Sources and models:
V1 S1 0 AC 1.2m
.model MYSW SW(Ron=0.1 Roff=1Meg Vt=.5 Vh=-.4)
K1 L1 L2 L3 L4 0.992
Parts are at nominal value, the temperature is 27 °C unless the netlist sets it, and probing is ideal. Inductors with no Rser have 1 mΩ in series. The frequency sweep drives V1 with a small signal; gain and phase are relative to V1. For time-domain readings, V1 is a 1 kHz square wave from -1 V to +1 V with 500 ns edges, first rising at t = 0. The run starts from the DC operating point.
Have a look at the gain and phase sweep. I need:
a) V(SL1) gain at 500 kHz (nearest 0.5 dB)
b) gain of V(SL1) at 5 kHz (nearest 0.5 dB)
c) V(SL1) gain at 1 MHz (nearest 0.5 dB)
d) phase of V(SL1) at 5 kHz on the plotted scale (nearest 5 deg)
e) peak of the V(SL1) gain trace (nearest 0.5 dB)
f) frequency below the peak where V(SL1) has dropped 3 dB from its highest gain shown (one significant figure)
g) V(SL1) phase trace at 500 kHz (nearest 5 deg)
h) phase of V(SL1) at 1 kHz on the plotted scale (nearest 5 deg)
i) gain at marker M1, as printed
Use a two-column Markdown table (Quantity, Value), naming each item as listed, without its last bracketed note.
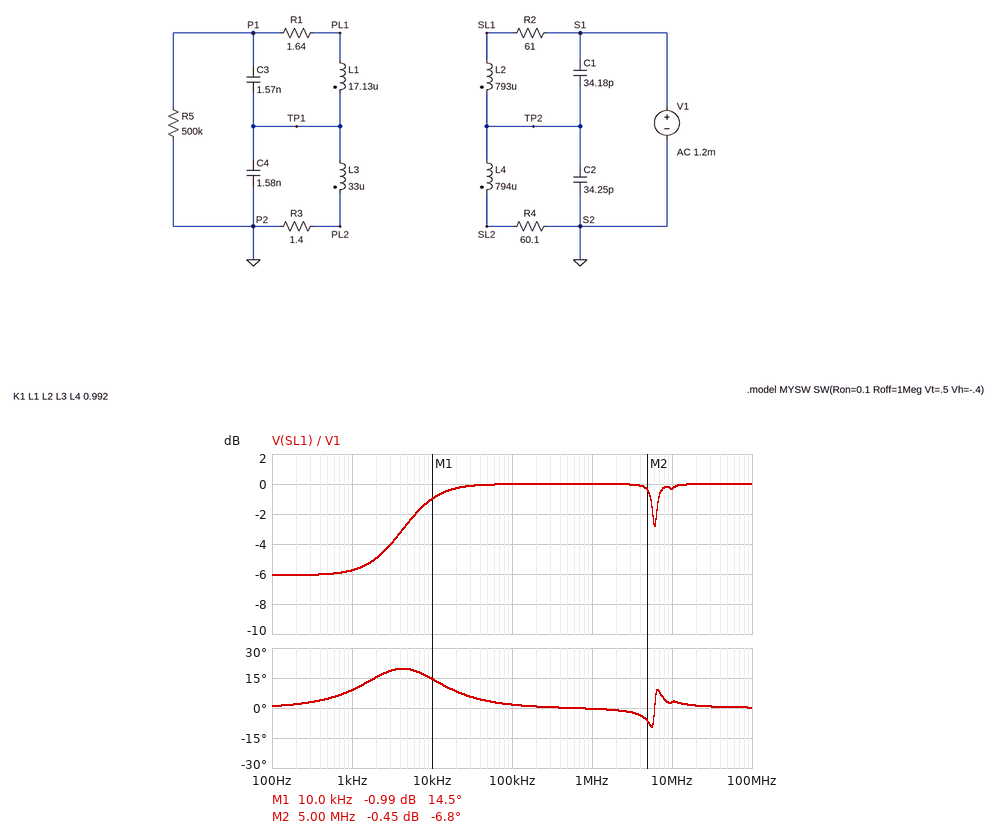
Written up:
| Quantity | Value |
|---|---|
| V(SL1) gain at 500 kHz | 0 dB |
| gain of V(SL1) at 5 kHz | -2.5 dB |
| V(SL1) gain at 1 MHz | 0 dB |
| phase of V(SL1) at 5 kHz on the plotted scale | 20 deg |
| peak of the V(SL1) gain trace | 0 dB |
| frequency below the peak where V(SL1) has dropped 3 dB from its highest gain shown | 4 kHz |
| V(SL1) phase trace at 500 kHz | 0 deg |
| phase of V(SL1) at 1 kHz on the plotted scale | 10 deg |
| gain at marker M1, as printed | -0.99 dB |
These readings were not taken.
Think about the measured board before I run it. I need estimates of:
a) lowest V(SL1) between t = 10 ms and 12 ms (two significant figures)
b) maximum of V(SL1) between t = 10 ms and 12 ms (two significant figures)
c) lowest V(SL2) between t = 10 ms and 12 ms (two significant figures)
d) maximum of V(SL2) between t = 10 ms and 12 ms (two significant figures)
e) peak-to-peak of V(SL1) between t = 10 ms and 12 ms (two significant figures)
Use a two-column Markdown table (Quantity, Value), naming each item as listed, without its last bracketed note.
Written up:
| Quantity | Value |
|---|---|
| lowest V(SL1) between t = 10 ms and 12 ms | -1.5 V |
| maximum of V(SL1) between t = 10 ms and 12 ms | 1.5 V |
| lowest V(SL2) between t = 10 ms and 12 ms | -500 mV |
| maximum of V(SL2) between t = 10 ms and 12 ms | 500 mV |
| peak-to-peak of V(SL1) between t = 10 ms and 12 ms | 3.0 V |
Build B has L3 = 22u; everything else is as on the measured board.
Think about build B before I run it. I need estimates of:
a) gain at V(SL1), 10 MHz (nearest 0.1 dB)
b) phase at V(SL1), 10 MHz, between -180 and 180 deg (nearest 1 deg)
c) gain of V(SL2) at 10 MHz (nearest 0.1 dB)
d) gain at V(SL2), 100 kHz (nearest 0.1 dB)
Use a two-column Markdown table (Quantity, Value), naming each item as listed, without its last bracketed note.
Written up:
| Quantity | Value |
|---|---|
| gain at V(SL1), 10 MHz | -0.2 dB |
| phase at V(SL1), 10 MHz, between -180 and 180 deg | 4 deg |
| gain of V(SL2) at 10 MHz | -23.3 dB |
| gain at V(SL2), 100 kHz | -30.6 dB |
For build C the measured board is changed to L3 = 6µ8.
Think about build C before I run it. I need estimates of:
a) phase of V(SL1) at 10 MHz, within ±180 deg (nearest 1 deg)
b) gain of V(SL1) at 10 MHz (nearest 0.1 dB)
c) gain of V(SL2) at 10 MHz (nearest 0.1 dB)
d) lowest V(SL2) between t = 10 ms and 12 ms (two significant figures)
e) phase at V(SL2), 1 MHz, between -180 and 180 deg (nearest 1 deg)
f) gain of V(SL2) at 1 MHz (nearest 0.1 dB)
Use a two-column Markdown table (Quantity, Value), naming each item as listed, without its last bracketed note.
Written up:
| Quantity | Value |
|---|---|
| phase of V(SL1) at 10 MHz, within ±180 deg | 5 deg |
| gain of V(SL1) at 10 MHz | -0.5 dB |
| gain of V(SL2) at 10 MHz | -20.6 dB |
| lowest V(SL2) between t = 10 ms and 12 ms | -500 mV |
| phase at V(SL2), 1 MHz, between -180 and 180 deg | 87 deg |
| gain of V(SL2) at 1 MHz | -56.7 dB |
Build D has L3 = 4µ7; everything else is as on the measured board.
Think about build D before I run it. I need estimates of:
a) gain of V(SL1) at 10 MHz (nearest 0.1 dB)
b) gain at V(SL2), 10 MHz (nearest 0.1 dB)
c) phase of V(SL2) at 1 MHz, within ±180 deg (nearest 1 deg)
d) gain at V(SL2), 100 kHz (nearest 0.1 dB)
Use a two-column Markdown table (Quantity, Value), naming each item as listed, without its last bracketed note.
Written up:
| Quantity | Value |
|---|---|
| gain of V(SL1) at 10 MHz | -0.5 dB |
| gain at V(SL2), 10 MHz | -20.7 dB |
| phase of V(SL2) at 1 MHz, within ±180 deg | 86 deg |
| gain at V(SL2), 100 kHz | -30.5 dB |
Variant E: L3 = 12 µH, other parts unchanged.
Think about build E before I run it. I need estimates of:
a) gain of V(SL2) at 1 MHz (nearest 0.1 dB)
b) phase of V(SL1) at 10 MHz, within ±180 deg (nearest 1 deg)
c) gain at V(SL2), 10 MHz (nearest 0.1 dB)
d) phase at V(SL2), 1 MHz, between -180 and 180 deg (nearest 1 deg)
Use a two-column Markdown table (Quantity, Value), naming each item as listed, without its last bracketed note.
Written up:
| Quantity | Value |
|---|---|
| gain of V(SL2) at 1 MHz | -52.2 dB |
| phase of V(SL1) at 10 MHz, within ±180 deg | 5 deg |
| gain at V(SL2), 10 MHz | -20.5 dB |
| phase at V(SL2), 1 MHz, between -180 and 180 deg | 88 deg |
